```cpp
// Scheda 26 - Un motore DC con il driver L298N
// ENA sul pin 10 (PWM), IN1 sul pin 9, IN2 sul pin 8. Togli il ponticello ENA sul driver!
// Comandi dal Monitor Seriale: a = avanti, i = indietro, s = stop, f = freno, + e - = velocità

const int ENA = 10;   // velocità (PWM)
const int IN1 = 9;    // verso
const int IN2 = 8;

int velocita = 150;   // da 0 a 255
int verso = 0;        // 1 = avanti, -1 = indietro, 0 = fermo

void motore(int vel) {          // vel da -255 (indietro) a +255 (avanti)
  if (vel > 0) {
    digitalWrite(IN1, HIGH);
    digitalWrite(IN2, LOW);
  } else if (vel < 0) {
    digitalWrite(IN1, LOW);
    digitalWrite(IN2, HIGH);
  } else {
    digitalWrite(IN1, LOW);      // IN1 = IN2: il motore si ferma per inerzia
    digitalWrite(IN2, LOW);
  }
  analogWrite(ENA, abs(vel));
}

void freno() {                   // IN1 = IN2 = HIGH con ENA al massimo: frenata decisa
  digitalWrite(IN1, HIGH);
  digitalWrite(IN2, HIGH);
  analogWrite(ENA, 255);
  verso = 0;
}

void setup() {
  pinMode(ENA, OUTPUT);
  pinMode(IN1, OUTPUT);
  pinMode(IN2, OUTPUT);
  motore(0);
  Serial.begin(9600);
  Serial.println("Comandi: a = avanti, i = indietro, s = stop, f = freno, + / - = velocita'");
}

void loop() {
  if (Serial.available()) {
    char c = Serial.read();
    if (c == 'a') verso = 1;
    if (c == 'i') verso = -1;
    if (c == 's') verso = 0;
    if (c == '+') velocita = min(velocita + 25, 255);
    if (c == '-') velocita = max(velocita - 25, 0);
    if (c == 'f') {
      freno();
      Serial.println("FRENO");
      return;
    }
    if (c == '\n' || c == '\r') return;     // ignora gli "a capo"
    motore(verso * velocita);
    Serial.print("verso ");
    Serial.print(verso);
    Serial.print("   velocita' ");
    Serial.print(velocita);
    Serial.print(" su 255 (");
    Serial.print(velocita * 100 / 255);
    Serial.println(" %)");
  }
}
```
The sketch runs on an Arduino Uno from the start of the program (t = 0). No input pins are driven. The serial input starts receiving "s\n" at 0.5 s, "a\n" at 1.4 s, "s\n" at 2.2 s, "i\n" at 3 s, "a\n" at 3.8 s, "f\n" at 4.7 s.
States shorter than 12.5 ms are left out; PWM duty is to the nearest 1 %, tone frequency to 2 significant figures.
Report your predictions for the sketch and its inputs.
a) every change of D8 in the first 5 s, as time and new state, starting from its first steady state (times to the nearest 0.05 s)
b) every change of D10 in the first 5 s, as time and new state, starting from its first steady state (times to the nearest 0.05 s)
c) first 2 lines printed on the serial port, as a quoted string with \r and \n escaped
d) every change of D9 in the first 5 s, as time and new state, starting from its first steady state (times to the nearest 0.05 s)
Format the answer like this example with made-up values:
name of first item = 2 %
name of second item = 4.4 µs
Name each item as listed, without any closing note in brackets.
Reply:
every change of D8 in the first 5 s, as time and new state, starting from its first steady state = 0 s low; 3 s high; 3.8 s low; 4.7 s high
every change of D10 in the first 5 s, as time and new state, starting from its first steady state = 0 s low; 1.4 s PWM 59 %; 2.2 s low; 3 s PWM 59 %; 4.7 s high
first 2 lines printed on the serial port, as a quoted string with \r and \n escaped = "Comandi: a = avanti, i = indietro, s = stop, f = freno, + / - = velocita'\r\nverso 0   velocita' 150 su 255 (58 %)\r\n"
every change of D9 in the first 5 s, as time and new state, starting from its first steady state = 0 s low; 1.4 s high; 2.2 s low; 3.8 s high
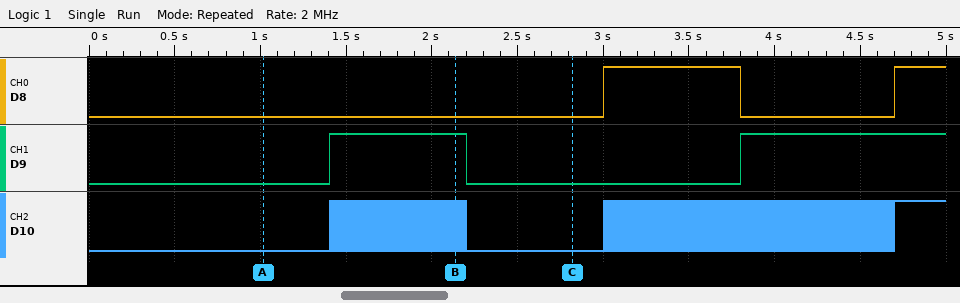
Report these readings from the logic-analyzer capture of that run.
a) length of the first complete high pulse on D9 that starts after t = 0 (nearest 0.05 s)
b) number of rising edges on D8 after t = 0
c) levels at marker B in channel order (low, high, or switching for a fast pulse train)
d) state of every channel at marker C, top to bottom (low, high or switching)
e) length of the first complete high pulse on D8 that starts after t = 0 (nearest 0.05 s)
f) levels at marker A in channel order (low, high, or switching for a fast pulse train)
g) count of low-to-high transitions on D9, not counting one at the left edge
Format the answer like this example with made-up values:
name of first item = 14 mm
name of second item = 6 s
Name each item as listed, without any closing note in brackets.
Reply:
length of the first complete high pulse on D9 that starts after t = 0 = 0.80 s
number of rising edges on D8 after t = 0 = 2
levels at marker B in channel order = D8 low, D9 high, D10 switching
state of every channel at marker C, top to bottom = D8 low, D9 low, D10 low
length of the first complete high pulse on D8 that starts after t = 0 = 0.80 s
levels at marker A in channel order = D8 low, D9 low, D10 low
count of low-to-high transitions on D9, not counting one at the left edge = 2
